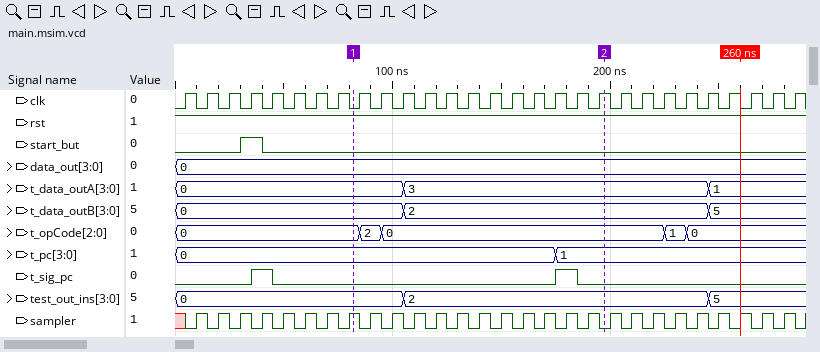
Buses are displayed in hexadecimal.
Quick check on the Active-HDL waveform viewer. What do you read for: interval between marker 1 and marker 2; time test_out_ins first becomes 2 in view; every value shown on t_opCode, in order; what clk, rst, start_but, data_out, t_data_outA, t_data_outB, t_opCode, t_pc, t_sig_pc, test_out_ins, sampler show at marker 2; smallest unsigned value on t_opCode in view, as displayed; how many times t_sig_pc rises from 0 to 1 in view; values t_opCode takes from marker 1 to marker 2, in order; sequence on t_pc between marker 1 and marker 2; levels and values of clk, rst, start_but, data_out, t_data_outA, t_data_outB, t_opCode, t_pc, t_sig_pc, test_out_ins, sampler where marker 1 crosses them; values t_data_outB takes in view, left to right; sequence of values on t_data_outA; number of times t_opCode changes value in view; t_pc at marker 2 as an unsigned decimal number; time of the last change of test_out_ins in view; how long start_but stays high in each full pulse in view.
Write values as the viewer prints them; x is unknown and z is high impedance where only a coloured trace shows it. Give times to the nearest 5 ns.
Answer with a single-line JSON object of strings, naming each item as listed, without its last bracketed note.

{"interval between marker 1 and marker 2": "115 ns", "time test_out_ins first becomes 2 in view": "105 ns", "every value shown on t_opCode, in order": "0, 2, 0, 1, 0", "what clk, rst, start_but, data_out, t_data_outA, t_data_outB, t_opCode, t_pc, t_sig_pc, test_out_ins, sampler show at marker 2": "clk=1, rst=1, start_but=0, data_out=0, t_data_outA=3, t_data_outB=2, t_opCode=0, t_pc=1, t_sig_pc=0, test_out_ins=2, sampler=0", "smallest unsigned value on t_opCode in view, as displayed": "0", "how many times t_sig_pc rises from 0 to 1 in view": "2", "values t_opCode takes from marker 1 to marker 2, in order": "0, 2, 0", "sequence on t_pc between marker 1 and marker 2": "0, 1", "levels and values of clk, rst, start_but, data_out, t_data_outA, t_data_outB, t_opCode, t_pc, t_sig_pc, test_out_ins, sampler where marker 1 crosses them": "clk=0, rst=1, start_but=0, data_out=0, t_data_outA=0, t_data_outB=0, t_opCode=0, t_pc=0, t_sig_pc=0, test_out_ins=0, sampler=1", "values t_data_outB takes in view, left to right": "0, 2, 5", "sequence of values on t_data_outA": "0, 3, 1", "number of times t_opCode changes value in view": "4", "t_pc at marker 2 as an unsigned decimal number": "1", "time of the last change of test_out_ins in view": "245 ns", "how long start_but stays high in each full pulse in view": "10 ns"}
